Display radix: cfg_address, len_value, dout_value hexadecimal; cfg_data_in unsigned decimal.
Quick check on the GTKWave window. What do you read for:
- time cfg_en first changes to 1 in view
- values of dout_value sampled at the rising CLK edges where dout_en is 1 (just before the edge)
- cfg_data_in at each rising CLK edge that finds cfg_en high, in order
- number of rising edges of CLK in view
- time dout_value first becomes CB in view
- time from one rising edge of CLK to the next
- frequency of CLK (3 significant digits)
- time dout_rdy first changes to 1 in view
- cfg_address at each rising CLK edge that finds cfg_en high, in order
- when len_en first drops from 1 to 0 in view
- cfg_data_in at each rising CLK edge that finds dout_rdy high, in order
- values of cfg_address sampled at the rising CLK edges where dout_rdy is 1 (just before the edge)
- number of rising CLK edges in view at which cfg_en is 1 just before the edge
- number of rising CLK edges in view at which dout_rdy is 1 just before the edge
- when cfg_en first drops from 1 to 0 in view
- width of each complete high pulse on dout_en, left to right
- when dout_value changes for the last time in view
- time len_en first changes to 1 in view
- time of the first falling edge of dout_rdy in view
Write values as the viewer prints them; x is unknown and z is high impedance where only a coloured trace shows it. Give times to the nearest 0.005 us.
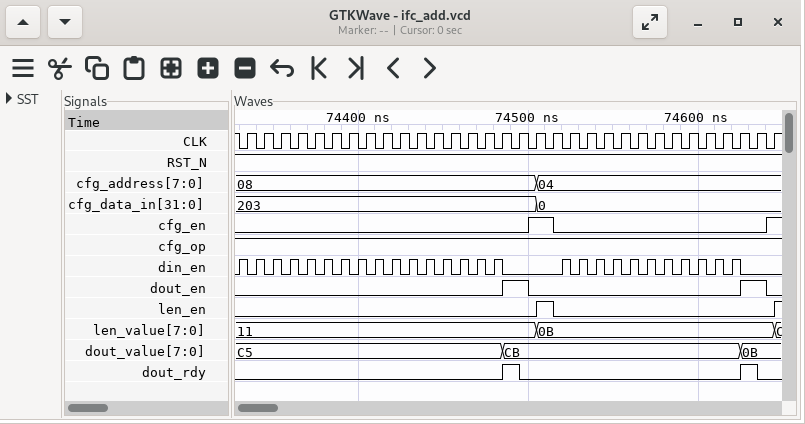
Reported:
74.5 us
CB, 0B
203, 0, 0
32
74.485 us
0.01 us
100 MHz
74.485 us
08, 04, 04
74.515 us
203, 0
08, 04
3
2
74.515 us
0.015 us, 0.015 us
74.625 us
74.505 us
74.495 us
